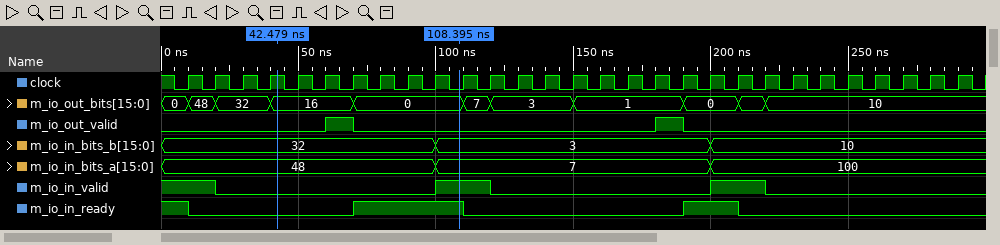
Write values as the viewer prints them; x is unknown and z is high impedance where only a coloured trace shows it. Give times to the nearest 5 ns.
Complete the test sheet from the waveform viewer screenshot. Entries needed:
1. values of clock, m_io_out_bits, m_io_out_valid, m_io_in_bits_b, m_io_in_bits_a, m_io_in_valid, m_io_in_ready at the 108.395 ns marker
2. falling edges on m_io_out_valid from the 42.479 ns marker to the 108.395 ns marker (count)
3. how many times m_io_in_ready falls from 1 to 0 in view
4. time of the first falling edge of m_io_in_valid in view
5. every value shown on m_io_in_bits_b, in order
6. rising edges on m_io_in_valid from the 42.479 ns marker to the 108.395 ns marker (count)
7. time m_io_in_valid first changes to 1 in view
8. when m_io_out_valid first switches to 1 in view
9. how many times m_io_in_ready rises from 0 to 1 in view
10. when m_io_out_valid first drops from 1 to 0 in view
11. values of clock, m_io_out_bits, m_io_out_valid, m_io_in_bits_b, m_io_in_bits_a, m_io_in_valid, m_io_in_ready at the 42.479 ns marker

clock=0, m_io_out_bits=0, m_io_out_valid=0, m_io_in_bits_b=3, m_io_in_bits_a=7, m_io_in_valid=1, m_io_in_ready=1
1
3
20 ns
32, 3, 10
1
100 ns
60 ns
2
70 ns
clock=1, m_io_out_bits=16, m_io_out_valid=0, m_io_in_bits_b=32, m_io_in_bits_a=48, m_io_in_valid=0, m_io_in_ready=0
